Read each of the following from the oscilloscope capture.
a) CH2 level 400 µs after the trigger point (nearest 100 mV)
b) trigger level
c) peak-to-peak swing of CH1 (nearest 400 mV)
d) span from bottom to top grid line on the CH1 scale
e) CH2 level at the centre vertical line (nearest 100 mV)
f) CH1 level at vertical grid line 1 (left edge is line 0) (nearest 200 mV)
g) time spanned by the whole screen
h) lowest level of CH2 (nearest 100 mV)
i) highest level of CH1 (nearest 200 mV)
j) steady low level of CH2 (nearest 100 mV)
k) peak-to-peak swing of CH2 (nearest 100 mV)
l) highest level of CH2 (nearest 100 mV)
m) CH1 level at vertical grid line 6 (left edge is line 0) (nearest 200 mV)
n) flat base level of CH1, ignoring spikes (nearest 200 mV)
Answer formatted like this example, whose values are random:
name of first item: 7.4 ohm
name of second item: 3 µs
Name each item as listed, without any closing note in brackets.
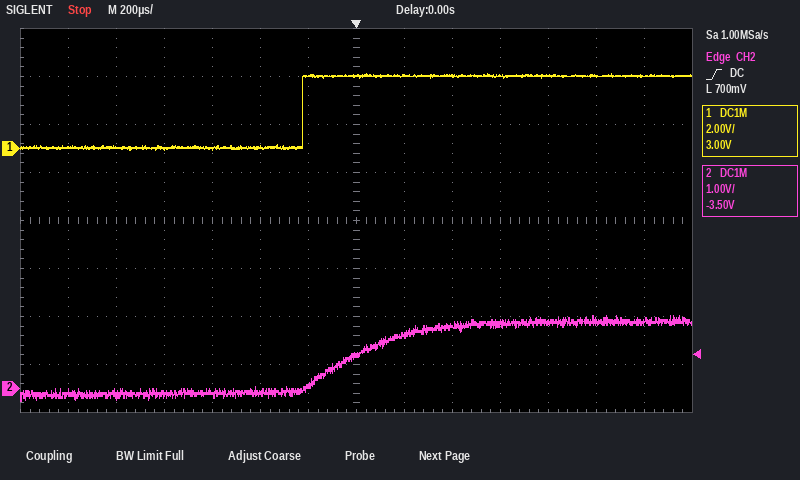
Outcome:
CH2 level 400 µs after the trigger point: 1.3 V
trigger level: 700 mV
peak-to-peak swing of CH1: 3.2 V
span from bottom to top grid line on the CH1 scale: 16 V
CH2 level at the centre vertical line: 700 mV
CH1 level at vertical grid line 1 (left edge is line 0): 0.0 V
time spanned by the whole screen: 2.8 ms
lowest level of CH2: -300 mV
highest level of CH1: 3.2 V
steady low level of CH2: -100 mV
peak-to-peak swing of CH2: 1.8 V
highest level of CH2: 1.5 V
CH1 level at vertical grid line 6 (left edge is line 0): 3.0 V
flat base level of CH1, ignoring spikes: 0.0 V
